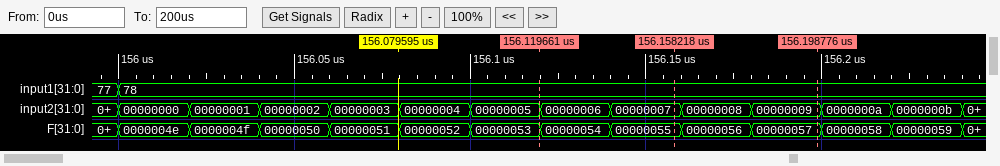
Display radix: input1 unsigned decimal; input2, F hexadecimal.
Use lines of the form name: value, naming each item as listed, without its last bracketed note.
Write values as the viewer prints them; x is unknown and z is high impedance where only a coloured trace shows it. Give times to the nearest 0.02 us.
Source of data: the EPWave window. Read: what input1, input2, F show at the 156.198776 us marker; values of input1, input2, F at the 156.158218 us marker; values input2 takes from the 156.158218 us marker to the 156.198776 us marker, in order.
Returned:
what input1, input2, F show at the 156.198776 us marker: input1=78, input2=00000009, F=00000057
values of input1, input2, F at the 156.158218 us marker: input1=78, input2=00000007, F=00000055
values input2 takes from the 156.158218 us marker to the 156.198776 us marker, in order: 00000007, 00000008, 00000009
